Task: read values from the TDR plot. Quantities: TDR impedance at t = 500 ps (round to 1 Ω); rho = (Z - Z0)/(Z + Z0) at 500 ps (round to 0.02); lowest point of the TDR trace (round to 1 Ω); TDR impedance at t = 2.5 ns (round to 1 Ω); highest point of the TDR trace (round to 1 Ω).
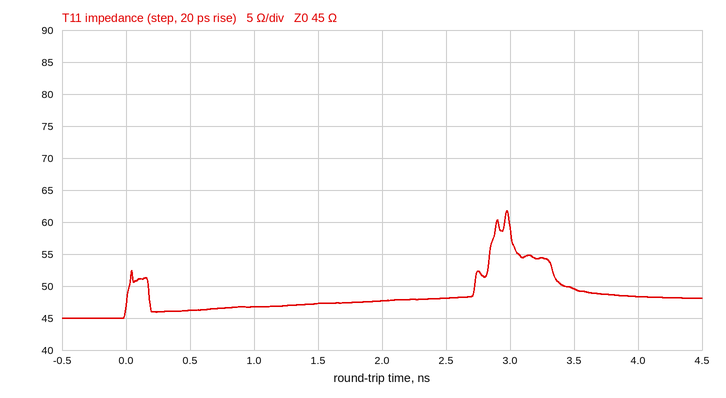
46 Ω
+0.02
45 Ω
48 Ω
62 Ω
